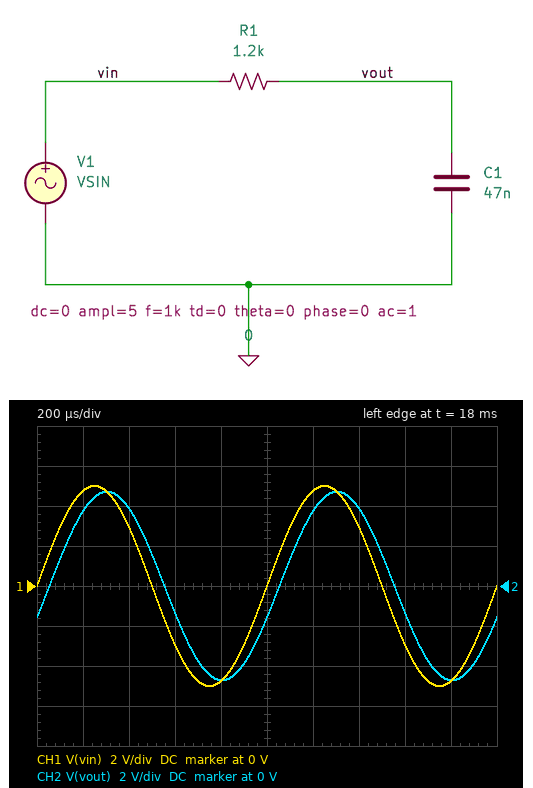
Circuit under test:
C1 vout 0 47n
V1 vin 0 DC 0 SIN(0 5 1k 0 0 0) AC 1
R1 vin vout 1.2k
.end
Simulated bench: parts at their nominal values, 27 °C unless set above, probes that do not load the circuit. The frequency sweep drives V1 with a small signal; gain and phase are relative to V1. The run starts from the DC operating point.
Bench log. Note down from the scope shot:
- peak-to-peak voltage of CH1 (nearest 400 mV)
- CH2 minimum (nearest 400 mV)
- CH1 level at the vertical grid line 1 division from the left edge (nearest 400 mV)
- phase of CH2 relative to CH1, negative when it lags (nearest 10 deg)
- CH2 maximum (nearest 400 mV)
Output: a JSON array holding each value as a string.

["10.0 V", "-4.8 V", "4.8 V", "-20 deg", "4.8 V"]
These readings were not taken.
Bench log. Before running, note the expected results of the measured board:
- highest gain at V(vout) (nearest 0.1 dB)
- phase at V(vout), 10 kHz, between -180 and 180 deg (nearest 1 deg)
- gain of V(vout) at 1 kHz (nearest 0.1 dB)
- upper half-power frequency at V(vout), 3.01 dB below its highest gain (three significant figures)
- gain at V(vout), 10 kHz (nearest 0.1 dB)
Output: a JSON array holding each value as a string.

["0 dB", "-74 deg", "-0.5 dB", "2.82 kHz", "-11.3 dB"]
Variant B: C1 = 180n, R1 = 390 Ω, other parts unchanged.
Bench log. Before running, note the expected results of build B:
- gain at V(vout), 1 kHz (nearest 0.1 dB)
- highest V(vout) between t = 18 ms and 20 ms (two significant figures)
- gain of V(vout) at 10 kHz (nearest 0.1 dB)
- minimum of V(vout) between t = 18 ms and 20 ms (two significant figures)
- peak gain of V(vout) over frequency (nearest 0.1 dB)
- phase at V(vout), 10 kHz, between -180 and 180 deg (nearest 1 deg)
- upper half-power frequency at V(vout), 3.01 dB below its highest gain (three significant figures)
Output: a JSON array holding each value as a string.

["-0.8 dB", "4.6 V", "-13.1 dB", "-4.6 V", "0 dB", "-77 deg", "2.27 kHz"]
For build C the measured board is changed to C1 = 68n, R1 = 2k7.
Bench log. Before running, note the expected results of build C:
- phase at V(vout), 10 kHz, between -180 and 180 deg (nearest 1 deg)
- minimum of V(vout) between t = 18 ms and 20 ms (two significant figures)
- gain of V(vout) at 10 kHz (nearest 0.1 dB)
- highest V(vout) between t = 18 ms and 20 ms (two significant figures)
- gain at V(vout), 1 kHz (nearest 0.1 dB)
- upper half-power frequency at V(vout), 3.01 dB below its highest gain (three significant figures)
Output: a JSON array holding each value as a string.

["-85 deg", "-3.3 V", "-21.3 dB", "3.3 V", "-3.7 dB", "867 Hz"]
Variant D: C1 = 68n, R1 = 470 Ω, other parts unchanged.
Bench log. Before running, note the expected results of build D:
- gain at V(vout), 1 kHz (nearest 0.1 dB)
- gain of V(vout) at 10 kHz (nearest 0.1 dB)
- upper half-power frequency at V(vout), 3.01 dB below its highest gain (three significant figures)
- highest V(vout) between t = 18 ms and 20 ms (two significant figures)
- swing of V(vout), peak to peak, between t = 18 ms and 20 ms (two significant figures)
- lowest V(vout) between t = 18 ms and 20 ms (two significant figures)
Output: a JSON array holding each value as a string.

["-0.2 dB", "-7.0 dB", "4.98 kHz", "4.9 V", "9.8 V", "-4.9 V"]
